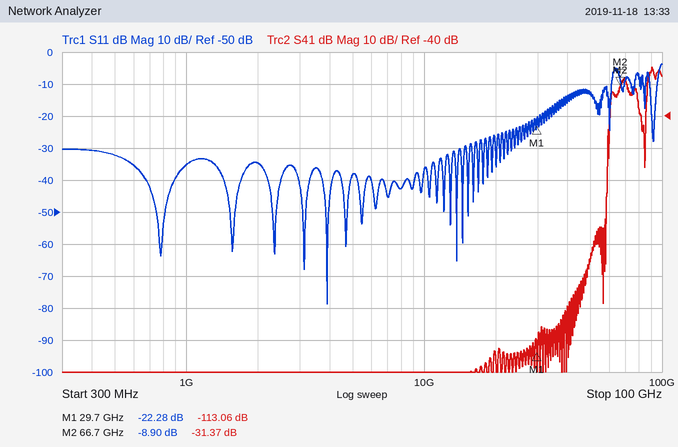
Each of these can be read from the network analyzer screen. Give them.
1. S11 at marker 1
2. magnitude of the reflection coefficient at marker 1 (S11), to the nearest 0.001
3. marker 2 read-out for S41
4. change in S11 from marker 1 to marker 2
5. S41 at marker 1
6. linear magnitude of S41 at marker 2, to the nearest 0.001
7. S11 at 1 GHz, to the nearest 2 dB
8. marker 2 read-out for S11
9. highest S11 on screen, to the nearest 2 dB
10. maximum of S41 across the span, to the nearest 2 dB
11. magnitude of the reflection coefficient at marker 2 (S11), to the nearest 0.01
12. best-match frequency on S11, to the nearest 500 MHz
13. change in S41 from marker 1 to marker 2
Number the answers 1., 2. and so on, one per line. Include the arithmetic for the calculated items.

1. -22.28 dB
2. 10^(-22.28/20) ≈ 0.077
3. -31.37 dB
4. -8.9 − (-22.28) = 13.38 dB
5. -113.06 dB
6. 10^(-31.37/20) ≈ 0.027
7. -36 dB
8. -8.90 dB
9. -4 dB
10. -24 dB
11. 10^(-8.9/20) ≈ 0.36
12. 4.0 GHz
13. -31.37 − (-113.06) = 81.69 dB
